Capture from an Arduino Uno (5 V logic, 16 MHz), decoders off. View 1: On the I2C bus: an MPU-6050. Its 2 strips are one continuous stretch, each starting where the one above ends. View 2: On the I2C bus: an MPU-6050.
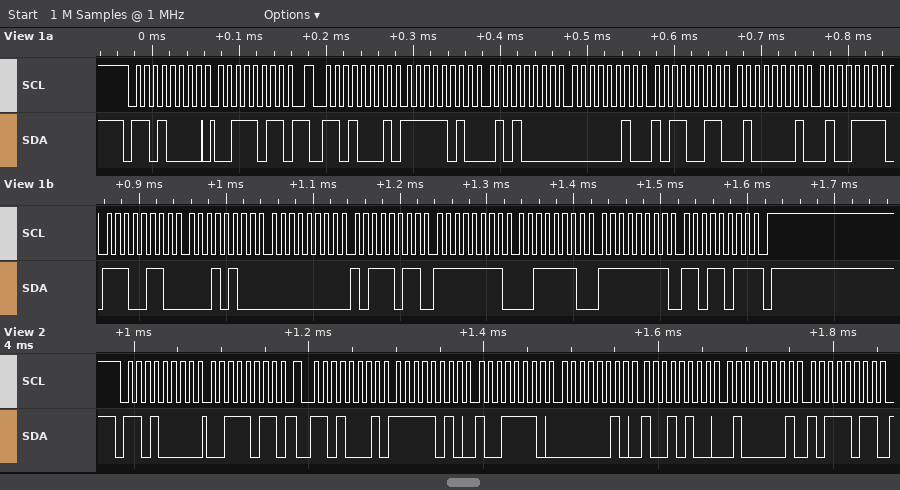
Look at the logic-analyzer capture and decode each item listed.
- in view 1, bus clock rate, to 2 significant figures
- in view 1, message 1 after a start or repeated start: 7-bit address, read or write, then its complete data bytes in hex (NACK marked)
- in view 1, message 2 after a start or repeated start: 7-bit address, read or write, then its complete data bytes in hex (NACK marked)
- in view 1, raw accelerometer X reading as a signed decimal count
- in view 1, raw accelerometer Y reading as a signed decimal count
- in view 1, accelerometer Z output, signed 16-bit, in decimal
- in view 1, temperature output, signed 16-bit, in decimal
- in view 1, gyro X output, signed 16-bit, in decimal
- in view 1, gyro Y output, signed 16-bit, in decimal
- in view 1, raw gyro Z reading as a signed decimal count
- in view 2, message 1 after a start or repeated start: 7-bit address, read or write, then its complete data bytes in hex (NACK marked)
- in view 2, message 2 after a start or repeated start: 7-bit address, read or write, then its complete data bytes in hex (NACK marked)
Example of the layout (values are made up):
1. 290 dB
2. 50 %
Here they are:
1. 100 kHz
2. 0x68 write: 3B
3. 0x68 read: FA 50 02 B3 41 4F E6 14 00 BB FF 3E FF DB NACK
4. -1456
5. 691
6. 16719
7. -6636
8. 187
9. -194
10. -37
11. 0x68 write: 3B
12. 0x68 read: FA 9E 02 94 41 BB
